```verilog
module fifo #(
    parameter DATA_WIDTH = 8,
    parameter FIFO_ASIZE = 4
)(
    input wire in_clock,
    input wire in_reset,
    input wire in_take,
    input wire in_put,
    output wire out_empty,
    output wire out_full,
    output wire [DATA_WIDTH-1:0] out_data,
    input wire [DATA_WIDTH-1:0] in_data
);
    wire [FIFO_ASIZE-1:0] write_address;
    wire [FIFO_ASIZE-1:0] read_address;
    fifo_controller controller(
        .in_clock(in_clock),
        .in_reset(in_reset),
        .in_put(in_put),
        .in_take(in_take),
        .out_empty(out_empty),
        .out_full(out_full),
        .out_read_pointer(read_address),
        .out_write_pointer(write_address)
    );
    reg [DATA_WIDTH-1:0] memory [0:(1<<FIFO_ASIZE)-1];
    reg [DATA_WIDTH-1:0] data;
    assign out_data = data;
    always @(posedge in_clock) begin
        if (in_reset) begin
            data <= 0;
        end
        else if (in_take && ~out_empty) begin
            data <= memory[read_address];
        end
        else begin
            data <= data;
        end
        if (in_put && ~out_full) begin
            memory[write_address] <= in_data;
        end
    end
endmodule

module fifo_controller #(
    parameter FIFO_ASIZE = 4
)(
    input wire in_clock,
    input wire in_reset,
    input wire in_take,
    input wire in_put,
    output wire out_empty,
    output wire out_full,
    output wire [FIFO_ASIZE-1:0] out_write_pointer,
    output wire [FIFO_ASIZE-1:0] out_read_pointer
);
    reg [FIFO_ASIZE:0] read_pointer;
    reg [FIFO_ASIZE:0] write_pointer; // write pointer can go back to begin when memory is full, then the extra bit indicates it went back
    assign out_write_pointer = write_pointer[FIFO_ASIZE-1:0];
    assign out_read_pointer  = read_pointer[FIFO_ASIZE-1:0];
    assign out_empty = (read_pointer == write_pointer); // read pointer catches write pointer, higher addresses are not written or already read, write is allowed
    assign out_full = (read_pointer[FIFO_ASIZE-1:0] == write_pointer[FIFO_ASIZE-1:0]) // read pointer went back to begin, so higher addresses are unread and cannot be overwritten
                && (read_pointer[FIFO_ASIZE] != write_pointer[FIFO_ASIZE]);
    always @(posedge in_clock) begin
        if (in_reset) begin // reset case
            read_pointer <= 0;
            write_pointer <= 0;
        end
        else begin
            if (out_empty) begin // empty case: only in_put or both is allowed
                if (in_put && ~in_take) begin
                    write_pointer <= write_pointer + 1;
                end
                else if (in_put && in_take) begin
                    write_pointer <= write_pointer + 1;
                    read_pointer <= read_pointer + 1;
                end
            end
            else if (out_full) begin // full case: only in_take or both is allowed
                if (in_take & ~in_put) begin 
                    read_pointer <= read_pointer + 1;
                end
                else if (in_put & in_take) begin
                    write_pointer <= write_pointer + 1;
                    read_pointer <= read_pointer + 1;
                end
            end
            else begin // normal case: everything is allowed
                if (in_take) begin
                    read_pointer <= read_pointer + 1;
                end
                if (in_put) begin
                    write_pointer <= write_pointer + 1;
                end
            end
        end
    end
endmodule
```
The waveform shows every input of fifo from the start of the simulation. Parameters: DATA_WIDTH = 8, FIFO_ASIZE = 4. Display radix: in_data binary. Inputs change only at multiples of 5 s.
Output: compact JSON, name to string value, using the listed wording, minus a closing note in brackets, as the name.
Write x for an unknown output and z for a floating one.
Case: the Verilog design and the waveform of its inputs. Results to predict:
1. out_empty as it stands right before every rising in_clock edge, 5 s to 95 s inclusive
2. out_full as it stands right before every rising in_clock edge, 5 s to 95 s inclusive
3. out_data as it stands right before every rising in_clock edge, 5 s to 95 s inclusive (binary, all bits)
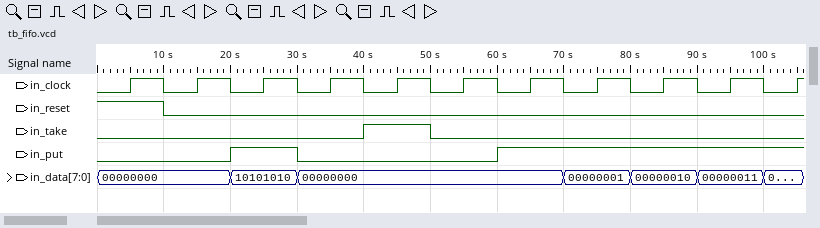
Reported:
{"out_empty as it stands right before every rising in_clock edge, 5 s to 95 s inclusive": "x 1 1 0 0 1 1 0 0 0", "out_full as it stands right before every rising in_clock edge, 5 s to 95 s inclusive": "x 0 0 0 0 0 0 0 0 0", "out_data as it stands right before every rising in_clock edge, 5 s to 95 s inclusive": "x, 00000000, 00000000, 00000000, 00000000, 10101010, 10101010, 10101010, 10101010, 10101010"}
